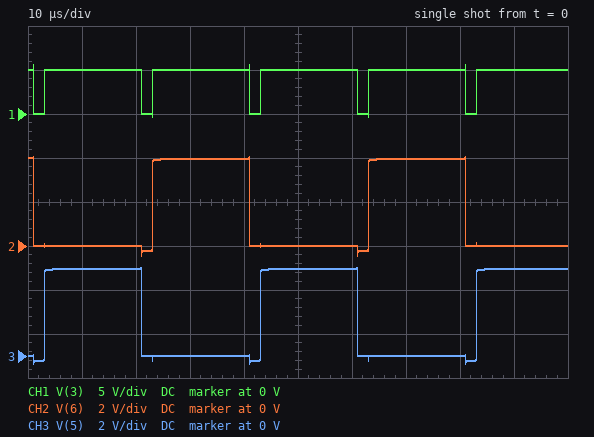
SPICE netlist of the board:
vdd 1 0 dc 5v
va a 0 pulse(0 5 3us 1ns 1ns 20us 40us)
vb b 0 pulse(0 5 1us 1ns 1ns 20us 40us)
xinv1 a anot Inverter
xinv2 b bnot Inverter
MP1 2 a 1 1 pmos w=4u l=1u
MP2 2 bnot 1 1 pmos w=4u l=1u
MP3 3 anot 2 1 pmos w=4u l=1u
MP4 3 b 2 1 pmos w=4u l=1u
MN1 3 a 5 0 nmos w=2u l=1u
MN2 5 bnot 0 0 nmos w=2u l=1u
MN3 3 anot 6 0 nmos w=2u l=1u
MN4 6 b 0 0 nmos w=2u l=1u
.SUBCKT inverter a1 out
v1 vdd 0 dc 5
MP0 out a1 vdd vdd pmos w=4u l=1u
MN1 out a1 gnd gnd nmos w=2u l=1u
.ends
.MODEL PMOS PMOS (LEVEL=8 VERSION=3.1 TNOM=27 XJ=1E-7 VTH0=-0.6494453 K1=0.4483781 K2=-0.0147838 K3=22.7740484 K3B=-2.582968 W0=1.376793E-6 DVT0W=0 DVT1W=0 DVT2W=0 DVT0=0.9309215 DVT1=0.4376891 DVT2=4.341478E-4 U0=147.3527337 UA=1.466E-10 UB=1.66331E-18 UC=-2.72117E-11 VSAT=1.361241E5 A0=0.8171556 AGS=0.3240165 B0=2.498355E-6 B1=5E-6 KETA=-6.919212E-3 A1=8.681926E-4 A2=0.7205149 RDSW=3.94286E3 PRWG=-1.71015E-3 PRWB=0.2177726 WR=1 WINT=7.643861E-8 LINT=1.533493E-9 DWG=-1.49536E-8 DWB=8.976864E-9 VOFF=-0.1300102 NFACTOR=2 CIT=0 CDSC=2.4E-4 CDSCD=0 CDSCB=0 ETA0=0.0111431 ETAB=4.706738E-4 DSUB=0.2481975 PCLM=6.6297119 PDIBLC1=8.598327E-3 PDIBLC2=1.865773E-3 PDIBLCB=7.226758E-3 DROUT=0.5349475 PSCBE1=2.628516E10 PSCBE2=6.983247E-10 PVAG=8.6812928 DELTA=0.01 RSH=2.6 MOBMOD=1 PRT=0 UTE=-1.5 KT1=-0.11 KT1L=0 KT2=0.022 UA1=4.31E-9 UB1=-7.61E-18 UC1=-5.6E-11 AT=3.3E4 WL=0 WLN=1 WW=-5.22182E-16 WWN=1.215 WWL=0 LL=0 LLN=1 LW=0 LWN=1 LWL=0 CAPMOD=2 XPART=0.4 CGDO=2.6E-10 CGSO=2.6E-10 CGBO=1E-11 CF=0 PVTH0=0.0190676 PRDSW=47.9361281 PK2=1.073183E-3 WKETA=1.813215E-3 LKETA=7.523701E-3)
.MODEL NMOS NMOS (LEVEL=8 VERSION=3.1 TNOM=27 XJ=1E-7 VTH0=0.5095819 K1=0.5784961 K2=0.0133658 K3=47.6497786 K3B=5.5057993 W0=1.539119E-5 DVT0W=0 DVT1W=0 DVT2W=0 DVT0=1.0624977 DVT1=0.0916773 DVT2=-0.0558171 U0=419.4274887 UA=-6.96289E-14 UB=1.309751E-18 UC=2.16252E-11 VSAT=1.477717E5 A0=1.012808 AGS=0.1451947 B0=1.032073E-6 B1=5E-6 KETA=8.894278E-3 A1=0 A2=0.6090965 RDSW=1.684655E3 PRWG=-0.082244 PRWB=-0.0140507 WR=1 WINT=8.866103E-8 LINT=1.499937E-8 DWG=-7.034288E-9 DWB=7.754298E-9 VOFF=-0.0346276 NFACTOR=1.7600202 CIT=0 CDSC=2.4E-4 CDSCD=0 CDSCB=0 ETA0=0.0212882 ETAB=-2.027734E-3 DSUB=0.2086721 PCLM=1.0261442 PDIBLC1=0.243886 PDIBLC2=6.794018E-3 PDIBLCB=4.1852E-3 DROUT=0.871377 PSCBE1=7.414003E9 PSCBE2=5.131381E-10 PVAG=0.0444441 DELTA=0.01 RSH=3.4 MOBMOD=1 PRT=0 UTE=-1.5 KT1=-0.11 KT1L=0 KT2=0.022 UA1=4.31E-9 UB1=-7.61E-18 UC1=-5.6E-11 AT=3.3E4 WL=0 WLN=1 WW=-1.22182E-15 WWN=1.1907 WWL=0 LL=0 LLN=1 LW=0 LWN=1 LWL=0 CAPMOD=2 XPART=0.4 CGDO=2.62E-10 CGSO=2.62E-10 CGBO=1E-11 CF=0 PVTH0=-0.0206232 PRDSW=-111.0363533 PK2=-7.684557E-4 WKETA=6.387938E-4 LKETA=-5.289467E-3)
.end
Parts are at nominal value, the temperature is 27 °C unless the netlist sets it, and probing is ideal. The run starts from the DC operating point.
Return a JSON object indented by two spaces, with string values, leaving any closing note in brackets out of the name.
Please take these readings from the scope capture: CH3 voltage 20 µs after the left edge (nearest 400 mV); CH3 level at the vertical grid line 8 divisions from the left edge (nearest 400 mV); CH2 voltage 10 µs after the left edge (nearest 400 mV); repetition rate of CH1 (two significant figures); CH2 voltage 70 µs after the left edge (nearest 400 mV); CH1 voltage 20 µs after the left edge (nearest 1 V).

{
  "CH3 voltage 20 µs after the left edge": "4.0 V",
  "CH3 level at the vertical grid line 8 divisions from the left edge": "0 V",
  "CH2 voltage 10 µs after the left edge": "0 V",
  "repetition rate of CH1": "50 kHz",
  "CH2 voltage 70 µs after the left edge": "4.0 V",
  "CH1 voltage 20 µs after the left edge": "5 V"
}
